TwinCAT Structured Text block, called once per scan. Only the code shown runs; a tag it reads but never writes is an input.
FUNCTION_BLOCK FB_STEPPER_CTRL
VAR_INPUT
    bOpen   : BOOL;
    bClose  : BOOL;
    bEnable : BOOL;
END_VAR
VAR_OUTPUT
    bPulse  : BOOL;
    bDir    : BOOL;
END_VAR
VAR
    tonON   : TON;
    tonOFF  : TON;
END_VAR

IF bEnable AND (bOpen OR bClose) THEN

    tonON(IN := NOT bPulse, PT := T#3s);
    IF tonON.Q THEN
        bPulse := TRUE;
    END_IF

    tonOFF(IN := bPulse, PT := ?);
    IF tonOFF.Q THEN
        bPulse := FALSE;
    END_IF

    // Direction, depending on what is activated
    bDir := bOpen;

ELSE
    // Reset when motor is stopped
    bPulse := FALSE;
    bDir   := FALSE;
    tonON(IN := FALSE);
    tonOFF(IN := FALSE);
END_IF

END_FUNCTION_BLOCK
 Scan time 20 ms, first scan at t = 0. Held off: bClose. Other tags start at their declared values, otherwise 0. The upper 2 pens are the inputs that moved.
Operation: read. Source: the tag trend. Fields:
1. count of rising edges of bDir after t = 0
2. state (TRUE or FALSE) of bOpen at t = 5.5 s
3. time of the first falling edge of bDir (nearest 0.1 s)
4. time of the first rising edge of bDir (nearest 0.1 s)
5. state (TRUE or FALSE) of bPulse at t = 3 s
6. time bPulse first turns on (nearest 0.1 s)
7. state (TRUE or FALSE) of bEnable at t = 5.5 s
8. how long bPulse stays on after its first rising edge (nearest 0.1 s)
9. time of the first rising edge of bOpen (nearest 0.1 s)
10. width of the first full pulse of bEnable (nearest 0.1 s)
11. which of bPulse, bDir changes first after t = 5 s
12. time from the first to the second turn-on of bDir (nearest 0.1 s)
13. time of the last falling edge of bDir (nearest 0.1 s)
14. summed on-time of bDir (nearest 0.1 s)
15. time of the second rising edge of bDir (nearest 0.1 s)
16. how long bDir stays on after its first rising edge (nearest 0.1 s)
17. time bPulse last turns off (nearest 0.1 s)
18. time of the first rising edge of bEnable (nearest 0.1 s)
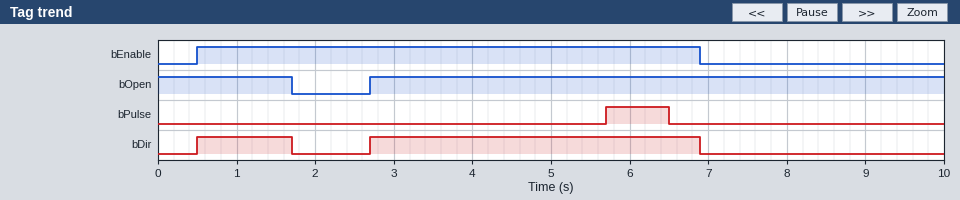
2
TRUE
1.7 s
0.5 s
FALSE
5.7 s
TRUE
0.8 s
2.7 s
6.4 s
bPulse
2.2 s
6.9 s
5.4 s
2.7 s
1.2 s
6.5 s
0.5 s
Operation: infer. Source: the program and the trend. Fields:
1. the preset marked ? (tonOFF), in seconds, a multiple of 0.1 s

0.8 s
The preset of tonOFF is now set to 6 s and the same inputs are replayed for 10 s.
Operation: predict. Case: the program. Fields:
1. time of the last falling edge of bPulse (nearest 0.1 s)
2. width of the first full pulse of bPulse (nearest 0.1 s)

6.9 s
1.2 s
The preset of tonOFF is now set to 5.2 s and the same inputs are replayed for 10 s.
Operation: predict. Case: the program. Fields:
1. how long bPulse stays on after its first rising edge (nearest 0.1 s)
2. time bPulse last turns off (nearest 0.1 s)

1.2 s
6.9 s
